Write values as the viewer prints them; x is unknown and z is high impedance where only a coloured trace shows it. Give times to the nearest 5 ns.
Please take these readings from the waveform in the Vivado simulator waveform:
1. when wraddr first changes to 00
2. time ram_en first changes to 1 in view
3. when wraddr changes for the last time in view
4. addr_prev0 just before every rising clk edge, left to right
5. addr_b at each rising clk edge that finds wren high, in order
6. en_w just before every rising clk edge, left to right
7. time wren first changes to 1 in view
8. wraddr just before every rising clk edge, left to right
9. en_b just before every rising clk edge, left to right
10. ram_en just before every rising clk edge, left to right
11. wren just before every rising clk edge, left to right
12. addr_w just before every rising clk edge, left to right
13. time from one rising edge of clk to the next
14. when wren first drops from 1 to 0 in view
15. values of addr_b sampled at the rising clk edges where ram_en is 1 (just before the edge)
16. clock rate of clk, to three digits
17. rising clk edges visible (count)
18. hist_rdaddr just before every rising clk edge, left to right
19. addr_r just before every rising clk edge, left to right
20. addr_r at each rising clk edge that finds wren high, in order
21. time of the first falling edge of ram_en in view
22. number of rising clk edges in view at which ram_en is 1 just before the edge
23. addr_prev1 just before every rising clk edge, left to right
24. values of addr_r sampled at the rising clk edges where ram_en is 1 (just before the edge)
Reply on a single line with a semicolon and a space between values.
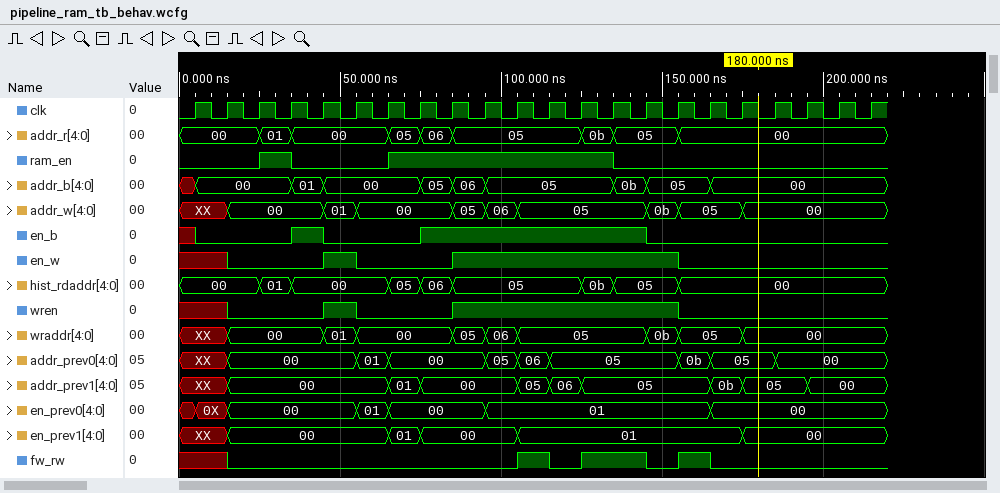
15 ns; 25 ns; 175 ns; XX, XX, 00, 00, 00, 00, 01, 00, 00, 00, 05, 06, 05, 05, 05, 05, 0b, 05, 05, 00, 00, 00; 00, 06, 05, 05, 05, 05, 0b, 05; x x 0 0 0 1 0 0 0 1 1 1 1 1 1 1 0 0 0 0 0 0; 45 ns; XX, XX, 00, 00, 00, 01, 00, 00, 00, 05, 06, 05, 05, 05, 05, 0b, 05, 05, 00, 00, 00, 00; x 0 0 0 1 0 0 0 1 1 1 1 1 1 1 0 0 0 0 0 0 0; 0 0 0 1 0 0 0 1 1 1 1 1 1 1 0 0 0 0 0 0 0 0; x x 0 0 0 1 0 0 0 1 1 1 1 1 1 1 0 0 0 0 0 0; XX, XX, 00, 00, 00, 01, 00, 00, 00, 05, 06, 05, 05, 05, 05, 0b, 05, 05, 00, 00, 00, 00; 10 ns; 55 ns; 00, 00, 05, 06, 05, 05, 05, 05; 100 MHz; 22; 00, 00, 00, 01, 00, 00, 00, 05, 06, 05, 05, 05, 05, 0b, 05, 05, 00, 00, 00, 00, 00, 00; 00, 00, 00, 01, 00, 00, 00, 05, 06, 05, 05, 05, 05, 0b, 05, 05, 00, 00, 00, 00, 00, 00; 00, 05, 05, 05, 05, 0b, 05, 05; 35 ns; 8; XX, XX, 00, 00, 00, 00, 00, 01, 00, 00, 00, 05, 06, 05, 05, 05, 05, 0b, 05, 05, 00, 00; 01, 05, 06, 05, 05, 05, 05, 0b
